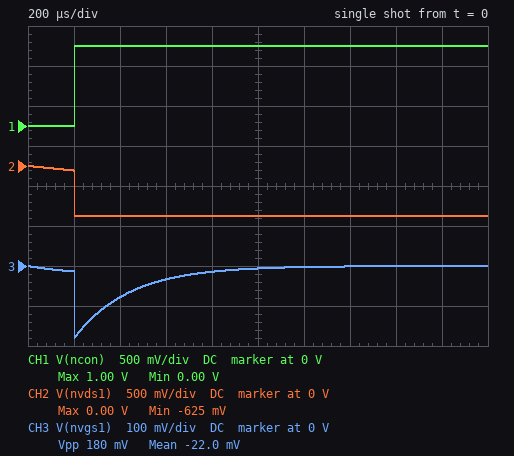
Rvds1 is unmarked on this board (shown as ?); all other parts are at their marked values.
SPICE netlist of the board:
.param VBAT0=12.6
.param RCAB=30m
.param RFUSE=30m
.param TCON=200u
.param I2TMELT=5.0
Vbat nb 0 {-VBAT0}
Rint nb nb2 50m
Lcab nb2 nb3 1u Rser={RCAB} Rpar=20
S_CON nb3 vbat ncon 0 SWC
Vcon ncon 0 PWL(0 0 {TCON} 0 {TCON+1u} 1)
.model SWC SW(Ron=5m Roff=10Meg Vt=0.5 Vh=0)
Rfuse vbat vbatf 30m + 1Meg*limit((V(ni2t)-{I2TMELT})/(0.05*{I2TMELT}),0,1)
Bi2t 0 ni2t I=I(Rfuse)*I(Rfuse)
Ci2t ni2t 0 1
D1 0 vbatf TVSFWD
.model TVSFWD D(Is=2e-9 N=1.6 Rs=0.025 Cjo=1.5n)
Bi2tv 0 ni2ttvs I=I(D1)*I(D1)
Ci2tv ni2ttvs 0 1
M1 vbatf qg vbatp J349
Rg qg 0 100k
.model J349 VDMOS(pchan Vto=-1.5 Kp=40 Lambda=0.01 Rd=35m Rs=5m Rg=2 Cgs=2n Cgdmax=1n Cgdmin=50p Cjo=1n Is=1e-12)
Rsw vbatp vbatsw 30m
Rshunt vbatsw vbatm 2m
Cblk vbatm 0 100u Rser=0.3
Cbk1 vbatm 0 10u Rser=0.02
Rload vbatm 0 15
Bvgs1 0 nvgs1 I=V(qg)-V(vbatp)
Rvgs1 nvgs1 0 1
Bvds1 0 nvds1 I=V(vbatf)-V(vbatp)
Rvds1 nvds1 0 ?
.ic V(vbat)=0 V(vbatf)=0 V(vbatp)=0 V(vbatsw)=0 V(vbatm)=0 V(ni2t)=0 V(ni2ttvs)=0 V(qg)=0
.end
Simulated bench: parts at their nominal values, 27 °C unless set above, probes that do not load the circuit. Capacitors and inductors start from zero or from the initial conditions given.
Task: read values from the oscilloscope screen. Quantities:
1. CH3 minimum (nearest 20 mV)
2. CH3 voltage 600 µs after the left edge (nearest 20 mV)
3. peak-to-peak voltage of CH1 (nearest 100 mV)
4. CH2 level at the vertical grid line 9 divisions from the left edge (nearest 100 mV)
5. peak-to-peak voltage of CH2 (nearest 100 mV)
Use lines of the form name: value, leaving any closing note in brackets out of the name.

CH3 minimum: -180 mV
CH3 voltage 600 µs after the left edge: -40 mV
peak-to-peak voltage of CH1: 1.0 V
CH2 level at the vertical grid line 9 divisions from the left edge: -600 mV
peak-to-peak voltage of CH2: 600 mV
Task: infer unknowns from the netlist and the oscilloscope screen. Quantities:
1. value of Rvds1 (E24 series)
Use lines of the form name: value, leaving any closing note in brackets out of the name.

value of Rvds1: 0.68 Ω
